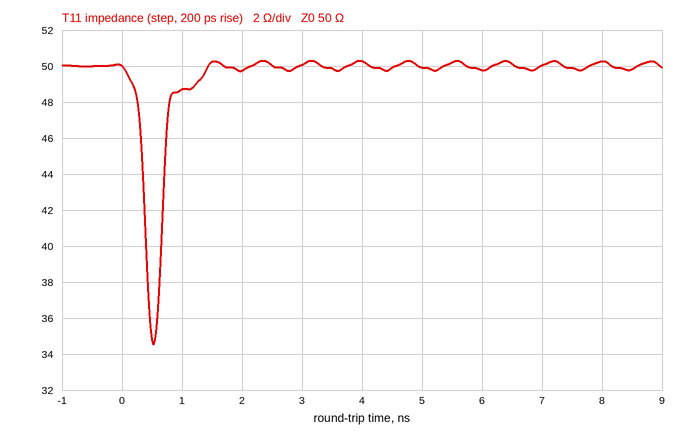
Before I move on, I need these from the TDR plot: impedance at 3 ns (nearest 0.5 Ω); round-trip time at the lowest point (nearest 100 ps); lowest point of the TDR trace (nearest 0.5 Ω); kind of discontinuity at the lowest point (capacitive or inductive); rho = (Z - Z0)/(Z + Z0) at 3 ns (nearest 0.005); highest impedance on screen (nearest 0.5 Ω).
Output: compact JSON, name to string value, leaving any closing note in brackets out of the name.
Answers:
{"impedance at 3 ns": "50.0 Ω", "round-trip time at the lowest point": "500 ps", "lowest point of the TDR trace": "34.5 Ω", "kind of discontinuity at the lowest point": "capacitive", "rho = (Z - Z0)/(Z + Z0) at 3 ns": "0.000", "highest impedance on screen": "50.5 Ω"}
